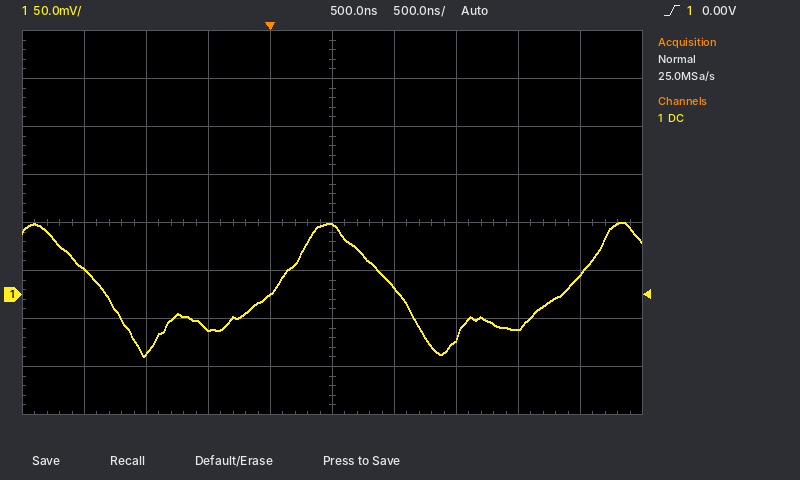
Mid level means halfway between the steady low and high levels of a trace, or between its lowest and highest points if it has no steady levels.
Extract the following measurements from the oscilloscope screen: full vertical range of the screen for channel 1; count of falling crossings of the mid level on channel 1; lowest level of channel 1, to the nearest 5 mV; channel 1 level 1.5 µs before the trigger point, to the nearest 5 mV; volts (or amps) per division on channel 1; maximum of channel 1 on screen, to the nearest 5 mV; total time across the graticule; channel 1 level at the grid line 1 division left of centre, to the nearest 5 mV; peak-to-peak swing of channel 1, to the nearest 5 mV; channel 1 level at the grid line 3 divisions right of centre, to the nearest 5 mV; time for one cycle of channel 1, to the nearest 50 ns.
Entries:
400 mV
2
-65 mV
25 mV
50 mV
75 mV
5 µs
0 mV
140 mV
-35 mV
2.35 µs
